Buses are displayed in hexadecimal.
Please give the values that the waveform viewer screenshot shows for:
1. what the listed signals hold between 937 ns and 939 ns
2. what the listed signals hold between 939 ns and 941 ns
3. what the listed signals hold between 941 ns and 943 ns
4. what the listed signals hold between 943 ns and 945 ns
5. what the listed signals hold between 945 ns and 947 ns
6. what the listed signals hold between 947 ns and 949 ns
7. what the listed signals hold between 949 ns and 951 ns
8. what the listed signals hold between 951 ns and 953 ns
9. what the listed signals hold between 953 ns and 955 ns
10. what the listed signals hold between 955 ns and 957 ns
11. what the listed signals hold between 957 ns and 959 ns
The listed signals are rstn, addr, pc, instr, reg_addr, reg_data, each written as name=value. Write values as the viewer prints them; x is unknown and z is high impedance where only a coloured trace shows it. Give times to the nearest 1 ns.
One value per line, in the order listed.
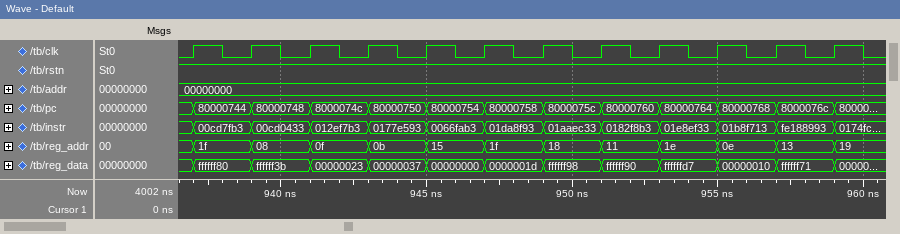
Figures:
rstn=1, addr=00000000, pc=80000744, instr=00cd7fb3, reg_addr=1f, reg_data=ffffff80
rstn=1, addr=00000000, pc=80000748, instr=00cd0433, reg_addr=08, reg_data=ffffff3b
rstn=1, addr=00000000, pc=8000074c, instr=012ef7b3, reg_addr=0f, reg_data=00000023
rstn=1, addr=00000000, pc=80000750, instr=0177e593, reg_addr=0b, reg_data=00000037
rstn=1, addr=00000000, pc=80000754, instr=0066fab3, reg_addr=15, reg_data=00000000
rstn=1, addr=00000000, pc=80000758, instr=01da8f93, reg_addr=1f, reg_data=0000001d
rstn=1, addr=00000000, pc=8000075c, instr=01aaec33, reg_addr=18, reg_data=ffffff98
rstn=1, addr=00000000, pc=80000760, instr=0182f8b3, reg_addr=11, reg_data=ffffff90
rstn=1, addr=00000000, pc=80000764, instr=01e8ef33, reg_addr=1e, reg_data=ffffffd7
rstn=1, addr=00000000, pc=80000768, instr=01b8f713, reg_addr=0e, reg_data=00000010
rstn=1, addr=00000000, pc=8000076c, instr=fe188993, reg_addr=13, reg_data=ffffff71
